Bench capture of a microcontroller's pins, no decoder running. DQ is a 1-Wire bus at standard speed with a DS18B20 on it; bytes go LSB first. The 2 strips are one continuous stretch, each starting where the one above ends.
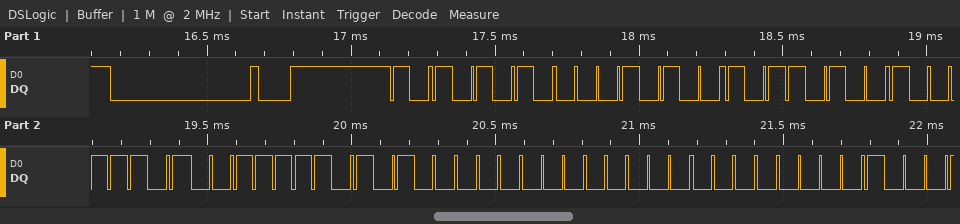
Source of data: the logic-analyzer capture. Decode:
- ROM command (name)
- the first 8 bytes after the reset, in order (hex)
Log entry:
Match ROM
55 28 2D B9 7C 05 00 00
